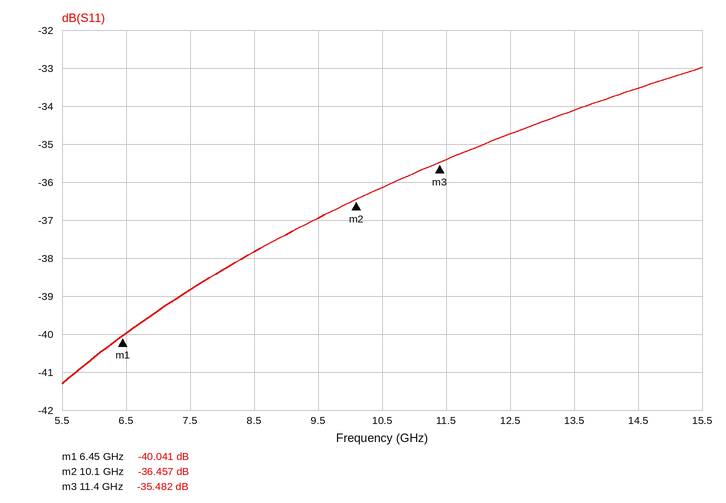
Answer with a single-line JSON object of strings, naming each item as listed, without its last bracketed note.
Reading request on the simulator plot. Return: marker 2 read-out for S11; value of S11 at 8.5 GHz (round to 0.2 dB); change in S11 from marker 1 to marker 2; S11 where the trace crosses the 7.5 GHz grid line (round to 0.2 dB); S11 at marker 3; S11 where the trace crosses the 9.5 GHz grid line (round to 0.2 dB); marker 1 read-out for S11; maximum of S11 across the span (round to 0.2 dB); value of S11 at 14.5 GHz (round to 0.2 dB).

{"marker 2 read-out for S11": "-36.457 dB", "value of S11 at 8.5 GHz": "-37.8 dB", "change in S11 from marker 1 to marker 2": "3.584 dB", "S11 where the trace crosses the 7.5 GHz grid line": "-38.8 dB", "S11 at marker 3": "-35.482 dB", "S11 where the trace crosses the 9.5 GHz grid line": "-37.0 dB", "marker 1 read-out for S11": "-40.041 dB", "maximum of S11 across the span": "-33.0 dB", "value of S11 at 14.5 GHz": "-33.6 dB"}
